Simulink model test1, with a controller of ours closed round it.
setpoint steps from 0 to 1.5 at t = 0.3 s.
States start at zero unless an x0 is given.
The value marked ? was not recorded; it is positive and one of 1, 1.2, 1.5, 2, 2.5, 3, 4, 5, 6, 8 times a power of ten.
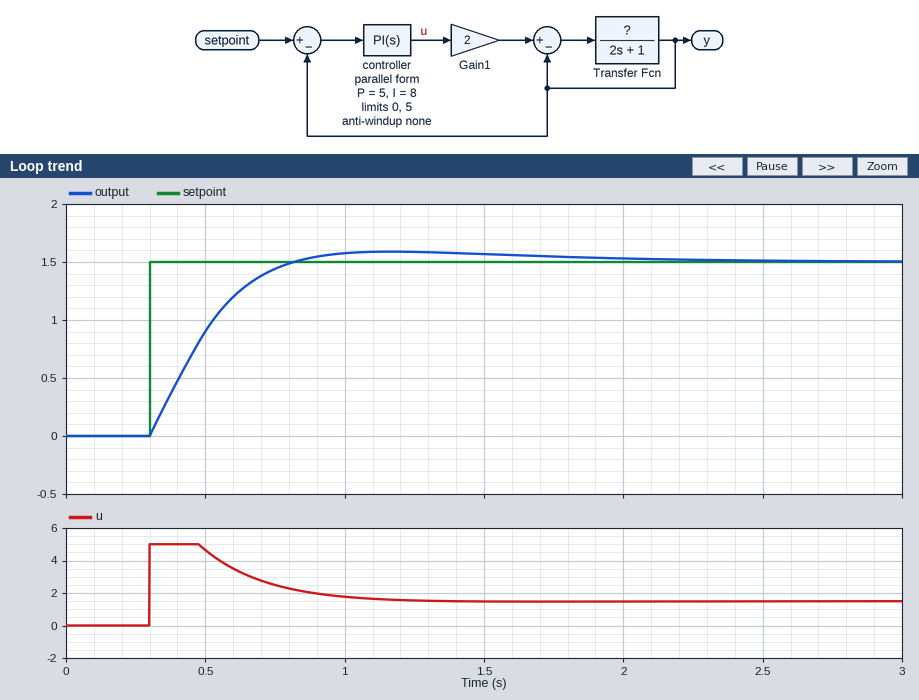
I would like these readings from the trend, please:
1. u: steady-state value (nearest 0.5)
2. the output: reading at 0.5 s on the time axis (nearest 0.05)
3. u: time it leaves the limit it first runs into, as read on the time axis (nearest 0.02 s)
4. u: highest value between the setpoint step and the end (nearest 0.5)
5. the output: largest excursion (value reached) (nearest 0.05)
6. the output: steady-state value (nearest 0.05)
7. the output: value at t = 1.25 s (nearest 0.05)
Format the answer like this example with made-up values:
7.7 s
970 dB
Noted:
1.5
0.90
0.48 s
5.0
1.60
1.50
1.60
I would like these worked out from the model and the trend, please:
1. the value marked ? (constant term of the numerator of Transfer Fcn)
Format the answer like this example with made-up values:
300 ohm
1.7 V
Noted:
1
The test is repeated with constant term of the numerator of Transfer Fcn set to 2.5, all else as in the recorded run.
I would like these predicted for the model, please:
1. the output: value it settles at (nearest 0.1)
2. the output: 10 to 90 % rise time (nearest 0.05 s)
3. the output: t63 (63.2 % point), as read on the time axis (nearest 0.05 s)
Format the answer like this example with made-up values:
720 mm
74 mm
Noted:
1.5
0.20 s
0.40 s
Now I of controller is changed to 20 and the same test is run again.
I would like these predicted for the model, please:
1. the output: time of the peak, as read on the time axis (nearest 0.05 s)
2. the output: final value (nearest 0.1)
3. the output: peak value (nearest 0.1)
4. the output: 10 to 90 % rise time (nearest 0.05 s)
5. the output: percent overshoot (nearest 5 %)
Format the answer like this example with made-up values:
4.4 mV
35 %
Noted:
0.90 s
1.5
1.9
0.30 s
25 %
